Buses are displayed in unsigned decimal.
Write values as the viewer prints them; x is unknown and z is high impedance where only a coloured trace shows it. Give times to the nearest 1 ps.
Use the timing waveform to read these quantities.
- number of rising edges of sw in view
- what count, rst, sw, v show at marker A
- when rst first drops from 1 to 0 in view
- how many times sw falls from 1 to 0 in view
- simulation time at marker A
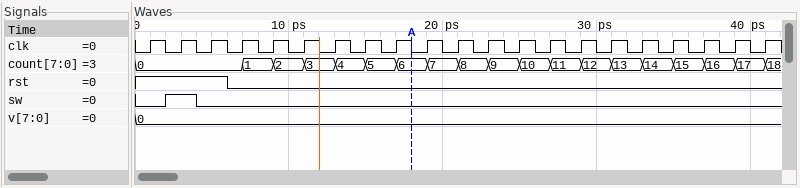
1
count=6, rst=0, sw=0, v=0
6 ps
1
18 ps
